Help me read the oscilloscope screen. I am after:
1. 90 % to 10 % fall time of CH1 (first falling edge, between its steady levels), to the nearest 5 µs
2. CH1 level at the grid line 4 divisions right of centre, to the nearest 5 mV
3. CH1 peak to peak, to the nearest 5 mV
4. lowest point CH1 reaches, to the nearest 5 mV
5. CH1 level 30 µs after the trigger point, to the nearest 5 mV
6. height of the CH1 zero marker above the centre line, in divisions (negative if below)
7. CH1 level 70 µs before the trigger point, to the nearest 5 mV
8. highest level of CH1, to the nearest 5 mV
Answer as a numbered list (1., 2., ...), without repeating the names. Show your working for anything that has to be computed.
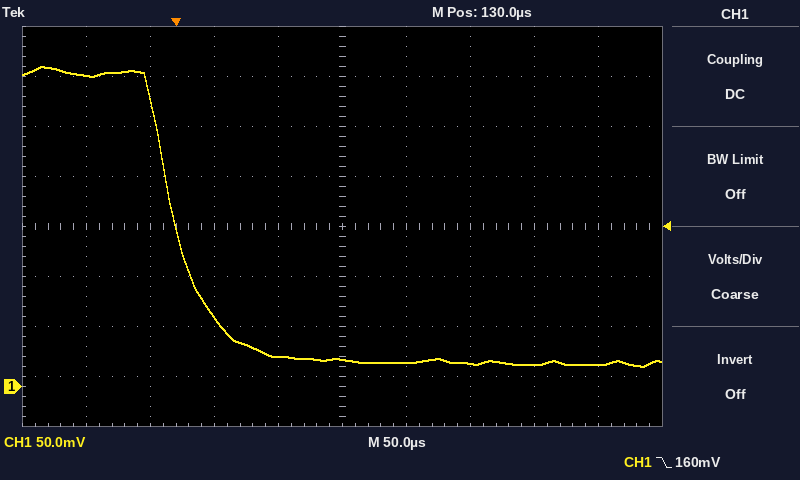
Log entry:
1. 60 µs
2. 20 mV
3. 320 mV − (20 mV) = 300 mV
4. 20 mV
5. 70 mV
6. -3.2 div
7. 310 mV
8. 320 mV
